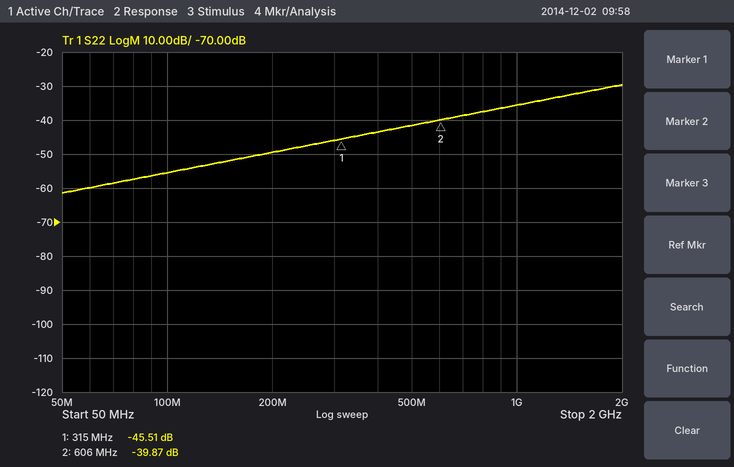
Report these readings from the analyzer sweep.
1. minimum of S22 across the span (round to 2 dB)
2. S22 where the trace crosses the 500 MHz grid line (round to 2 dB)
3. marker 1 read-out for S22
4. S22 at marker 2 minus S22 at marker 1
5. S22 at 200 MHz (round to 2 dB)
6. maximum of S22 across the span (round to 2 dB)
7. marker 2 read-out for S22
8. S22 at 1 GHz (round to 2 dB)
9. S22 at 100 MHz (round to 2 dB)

-62 dB
-42 dB
-45.51 dB
5.64 dB
-50 dB
-30 dB
-39.87 dB
-36 dB
-56 dB
